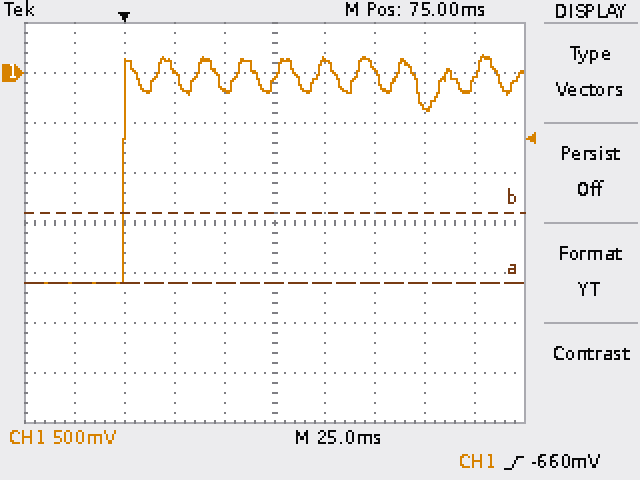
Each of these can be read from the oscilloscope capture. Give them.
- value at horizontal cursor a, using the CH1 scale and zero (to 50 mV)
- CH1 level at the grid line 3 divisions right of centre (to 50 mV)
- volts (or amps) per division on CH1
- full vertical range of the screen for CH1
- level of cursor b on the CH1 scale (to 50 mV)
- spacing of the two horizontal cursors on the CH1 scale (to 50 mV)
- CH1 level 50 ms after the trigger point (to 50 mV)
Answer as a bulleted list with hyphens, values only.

- -2.10 V
- -350 mV
- 500 mV
- 4 V
- -1.40 V
- 700 mV
- -150 mV
